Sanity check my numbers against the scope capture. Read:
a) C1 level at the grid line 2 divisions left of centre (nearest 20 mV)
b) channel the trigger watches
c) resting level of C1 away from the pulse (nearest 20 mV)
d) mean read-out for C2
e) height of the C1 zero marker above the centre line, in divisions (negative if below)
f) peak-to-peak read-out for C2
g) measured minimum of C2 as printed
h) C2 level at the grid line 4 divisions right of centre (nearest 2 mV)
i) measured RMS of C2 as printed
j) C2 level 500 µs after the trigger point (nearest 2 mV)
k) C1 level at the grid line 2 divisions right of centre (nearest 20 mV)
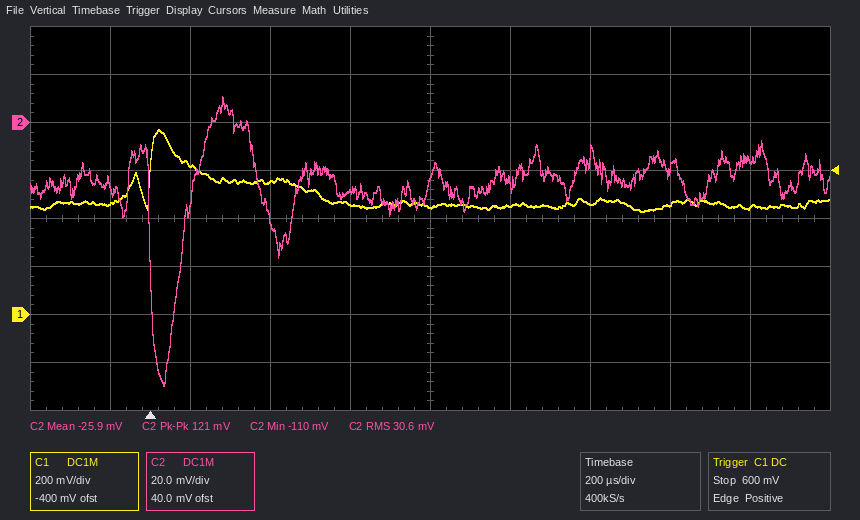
560 mV
C1
460 mV
-25.9 mV
-2.0 div
121 mV
-110 mV
-16 mV
30.6 mV
-28 mV
460 mV
